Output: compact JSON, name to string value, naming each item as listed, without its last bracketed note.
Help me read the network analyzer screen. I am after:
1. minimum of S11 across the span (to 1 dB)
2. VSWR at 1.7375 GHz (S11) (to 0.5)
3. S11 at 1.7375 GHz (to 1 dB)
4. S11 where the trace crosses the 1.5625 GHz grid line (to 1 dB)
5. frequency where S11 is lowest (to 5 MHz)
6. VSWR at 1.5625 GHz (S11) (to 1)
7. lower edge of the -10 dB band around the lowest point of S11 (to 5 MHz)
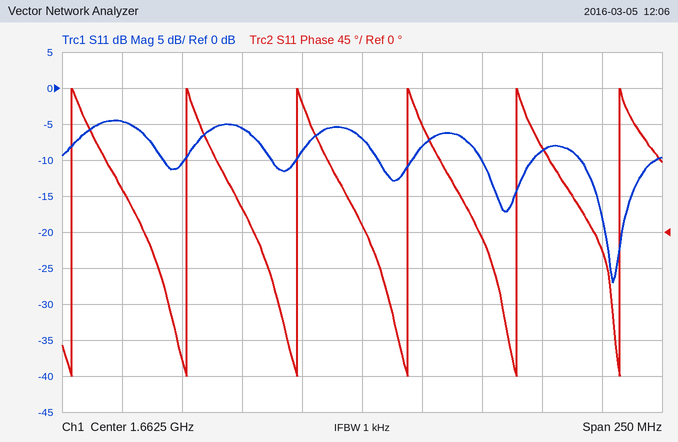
{"minimum of S11 across the span": "-27 dB", "VSWR at 1.7375 GHz (S11)": "2.0", "S11 at 1.7375 GHz": "-9 dB", "S11 where the trace crosses the 1.5625 GHz grid line": "-5 dB", "frequency where S11 is lowest": "1.765 GHz", "VSWR at 1.5625 GHz (S11)": "4", "lower edge of the -10 dB band around the lowest point of S11": "1.755 GHz"}
